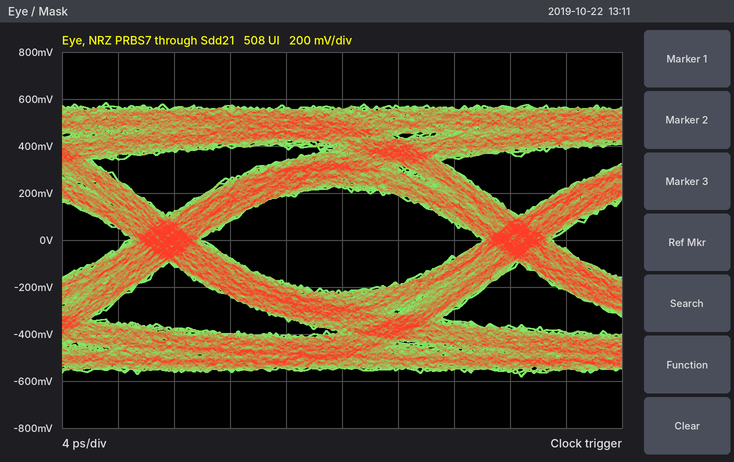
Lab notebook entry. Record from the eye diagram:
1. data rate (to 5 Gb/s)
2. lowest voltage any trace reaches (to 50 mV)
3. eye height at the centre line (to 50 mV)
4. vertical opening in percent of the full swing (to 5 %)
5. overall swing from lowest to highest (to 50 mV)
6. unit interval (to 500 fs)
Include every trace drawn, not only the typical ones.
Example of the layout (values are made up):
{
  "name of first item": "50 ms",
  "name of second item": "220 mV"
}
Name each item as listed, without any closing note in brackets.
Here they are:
{
  "data rate": "40 Gb/s",
  "lowest voltage any trace reaches": "-600 mV",
  "eye height at the centre line": "450 mV",
  "vertical opening in percent of the full swing": "40 %",
  "overall swing from lowest to highest": "1.15 V",
  "unit interval": "25.0 ps"
}
